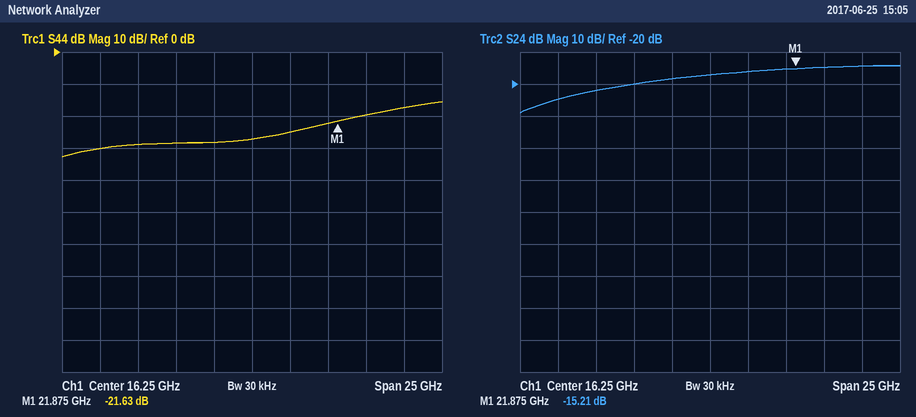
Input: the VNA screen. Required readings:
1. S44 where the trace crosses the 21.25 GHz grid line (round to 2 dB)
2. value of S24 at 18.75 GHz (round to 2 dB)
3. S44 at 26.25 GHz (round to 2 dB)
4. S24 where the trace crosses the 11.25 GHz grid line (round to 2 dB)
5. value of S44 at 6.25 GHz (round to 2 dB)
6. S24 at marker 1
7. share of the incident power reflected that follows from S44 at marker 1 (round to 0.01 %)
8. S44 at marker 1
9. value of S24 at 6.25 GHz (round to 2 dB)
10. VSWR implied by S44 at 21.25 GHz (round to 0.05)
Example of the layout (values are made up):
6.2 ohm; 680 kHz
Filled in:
-22 dB; -16 dB; -18 dB; -20 dB; -30 dB; -15.21 dB; 0.69 %; -21.63 dB; -24 dB; 1.15
